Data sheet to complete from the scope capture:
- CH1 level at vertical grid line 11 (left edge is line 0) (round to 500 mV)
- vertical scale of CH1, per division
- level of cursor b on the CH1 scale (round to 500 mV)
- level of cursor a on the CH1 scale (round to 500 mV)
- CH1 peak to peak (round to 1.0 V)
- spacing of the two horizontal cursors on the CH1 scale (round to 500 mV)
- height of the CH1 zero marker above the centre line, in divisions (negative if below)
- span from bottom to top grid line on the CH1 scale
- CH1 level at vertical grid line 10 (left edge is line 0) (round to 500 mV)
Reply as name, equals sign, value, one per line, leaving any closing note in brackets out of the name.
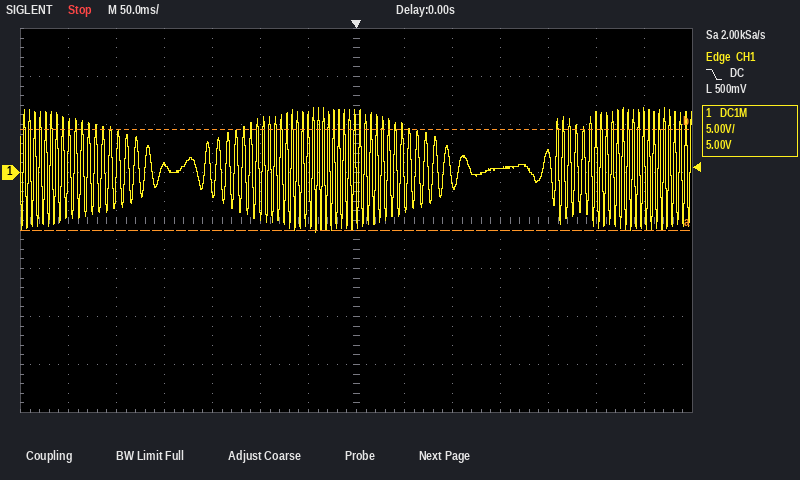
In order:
CH1 level at vertical grid line 11 (left edge is line 0) = 2.0 V
vertical scale of CH1, per division = 5 V
level of cursor b on the CH1 scale = 4.5 V
level of cursor a on the CH1 scale = -6.0 V
CH1 peak to peak = 13.0 V
spacing of the two horizontal cursors on the CH1 scale = 10.5 V
height of the CH1 zero marker above the centre line, in divisions = +1.0 div
span from bottom to top grid line on the CH1 scale = 40 V
CH1 level at vertical grid line 10 (left edge is line 0) = 500 mV
